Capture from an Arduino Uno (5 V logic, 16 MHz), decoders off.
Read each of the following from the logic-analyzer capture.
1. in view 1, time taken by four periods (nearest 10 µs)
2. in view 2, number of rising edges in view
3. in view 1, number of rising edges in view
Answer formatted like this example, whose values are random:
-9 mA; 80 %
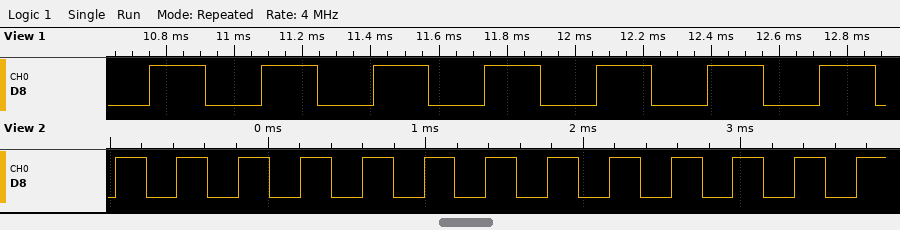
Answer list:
1310 µs; 13; 7
